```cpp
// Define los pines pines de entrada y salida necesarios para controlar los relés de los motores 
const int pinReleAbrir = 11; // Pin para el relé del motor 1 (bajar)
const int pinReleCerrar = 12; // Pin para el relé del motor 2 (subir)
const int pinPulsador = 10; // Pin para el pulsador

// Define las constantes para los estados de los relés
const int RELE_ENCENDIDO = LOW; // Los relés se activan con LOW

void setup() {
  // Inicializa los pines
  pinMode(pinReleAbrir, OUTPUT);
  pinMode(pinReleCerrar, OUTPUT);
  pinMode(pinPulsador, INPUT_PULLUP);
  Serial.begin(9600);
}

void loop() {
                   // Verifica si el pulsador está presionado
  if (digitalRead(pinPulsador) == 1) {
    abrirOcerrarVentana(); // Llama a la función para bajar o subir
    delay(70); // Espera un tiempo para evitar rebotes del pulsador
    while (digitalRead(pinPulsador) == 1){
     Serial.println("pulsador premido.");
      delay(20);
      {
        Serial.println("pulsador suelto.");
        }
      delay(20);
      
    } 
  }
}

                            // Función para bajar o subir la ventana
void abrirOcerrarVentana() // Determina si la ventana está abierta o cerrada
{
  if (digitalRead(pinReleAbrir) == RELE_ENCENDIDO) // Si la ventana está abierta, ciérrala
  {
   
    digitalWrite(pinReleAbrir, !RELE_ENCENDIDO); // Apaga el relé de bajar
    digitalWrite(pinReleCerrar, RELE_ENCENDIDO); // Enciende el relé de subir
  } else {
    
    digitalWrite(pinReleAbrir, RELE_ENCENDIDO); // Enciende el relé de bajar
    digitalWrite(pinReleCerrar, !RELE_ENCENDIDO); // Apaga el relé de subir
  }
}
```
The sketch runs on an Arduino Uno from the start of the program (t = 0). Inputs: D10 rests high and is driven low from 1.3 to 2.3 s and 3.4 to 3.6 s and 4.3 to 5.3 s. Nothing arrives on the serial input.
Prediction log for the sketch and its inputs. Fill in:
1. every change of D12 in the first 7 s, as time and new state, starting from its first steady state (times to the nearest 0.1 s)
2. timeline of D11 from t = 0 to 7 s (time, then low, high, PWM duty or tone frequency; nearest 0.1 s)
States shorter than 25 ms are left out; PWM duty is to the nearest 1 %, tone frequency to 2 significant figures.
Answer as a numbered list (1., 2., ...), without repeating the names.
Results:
1. 0 s low; 2.3 s high; 3.6 s low; 5.3 s high
2. 0 s high; 2.3 s low; 3.6 s high; 5.3 s low
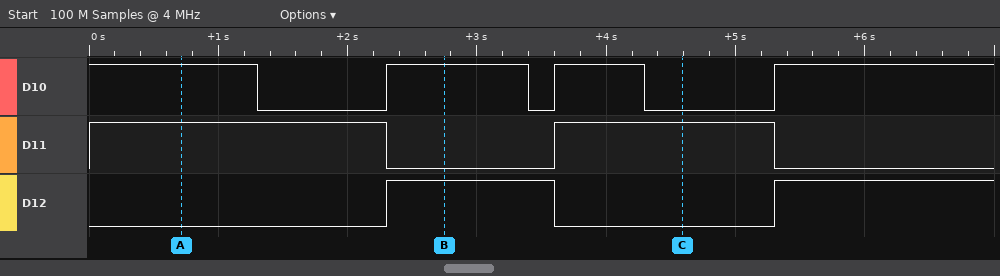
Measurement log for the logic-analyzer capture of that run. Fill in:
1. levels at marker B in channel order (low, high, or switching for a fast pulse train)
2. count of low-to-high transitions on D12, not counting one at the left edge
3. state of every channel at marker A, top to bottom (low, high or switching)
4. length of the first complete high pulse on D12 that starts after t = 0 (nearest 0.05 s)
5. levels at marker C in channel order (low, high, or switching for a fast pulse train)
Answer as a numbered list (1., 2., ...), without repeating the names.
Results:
1. D10 high, D11 low, D12 high
2. 2
3. D10 high, D11 high, D12 low
4. 1.30 s
5. D10 low, D11 high, D12 low
